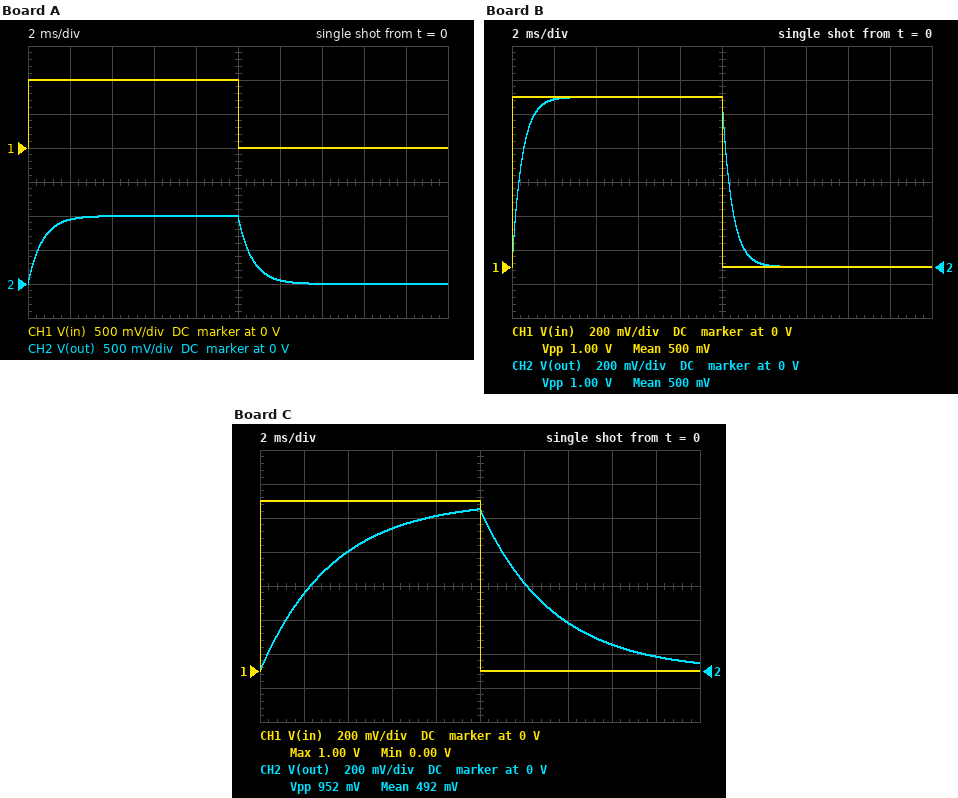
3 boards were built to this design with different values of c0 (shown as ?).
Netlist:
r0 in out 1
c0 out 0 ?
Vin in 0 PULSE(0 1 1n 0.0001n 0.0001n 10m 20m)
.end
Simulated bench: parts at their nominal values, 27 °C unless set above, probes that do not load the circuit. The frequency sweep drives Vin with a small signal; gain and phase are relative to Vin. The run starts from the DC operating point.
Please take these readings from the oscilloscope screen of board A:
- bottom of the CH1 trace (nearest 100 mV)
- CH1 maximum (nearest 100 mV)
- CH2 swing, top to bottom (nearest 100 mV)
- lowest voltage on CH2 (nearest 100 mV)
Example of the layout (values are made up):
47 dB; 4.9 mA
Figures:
0 V; 1.0 V; 1.0 V; 0 V
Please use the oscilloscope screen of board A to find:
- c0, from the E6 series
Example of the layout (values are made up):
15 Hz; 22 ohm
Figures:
680 µF
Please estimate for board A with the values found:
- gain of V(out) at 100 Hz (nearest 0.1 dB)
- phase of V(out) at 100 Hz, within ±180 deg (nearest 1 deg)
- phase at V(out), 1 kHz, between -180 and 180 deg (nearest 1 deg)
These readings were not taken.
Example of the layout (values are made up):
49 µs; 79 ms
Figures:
-0.7 dB; -23 deg; -77 deg
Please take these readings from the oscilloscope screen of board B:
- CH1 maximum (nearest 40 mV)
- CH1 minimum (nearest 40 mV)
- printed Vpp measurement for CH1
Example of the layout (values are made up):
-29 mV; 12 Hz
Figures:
1.00 V; 0 V; 1.00 V
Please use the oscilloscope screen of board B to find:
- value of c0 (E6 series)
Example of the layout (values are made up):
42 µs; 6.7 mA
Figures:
470 µF
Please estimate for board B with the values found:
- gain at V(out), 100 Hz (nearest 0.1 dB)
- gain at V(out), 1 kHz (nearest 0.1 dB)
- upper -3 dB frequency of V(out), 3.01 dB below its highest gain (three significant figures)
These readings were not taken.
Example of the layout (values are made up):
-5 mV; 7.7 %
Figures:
-0.4 dB; -9.9 dB; 339 Hz
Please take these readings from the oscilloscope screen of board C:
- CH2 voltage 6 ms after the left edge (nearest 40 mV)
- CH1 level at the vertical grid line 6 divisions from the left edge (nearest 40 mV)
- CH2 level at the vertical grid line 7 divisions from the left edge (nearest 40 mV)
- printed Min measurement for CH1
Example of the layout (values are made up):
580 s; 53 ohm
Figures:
840 mV; 0 V; 280 mV; 0.00 V
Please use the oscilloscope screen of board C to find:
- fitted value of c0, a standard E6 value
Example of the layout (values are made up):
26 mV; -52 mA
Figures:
3.3 mF
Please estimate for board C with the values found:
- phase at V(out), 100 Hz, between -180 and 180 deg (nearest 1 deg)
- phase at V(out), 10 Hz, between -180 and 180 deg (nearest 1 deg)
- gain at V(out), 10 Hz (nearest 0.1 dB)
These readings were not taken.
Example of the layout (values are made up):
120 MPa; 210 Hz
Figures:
-64 deg; -12 deg; -0.2 dB
